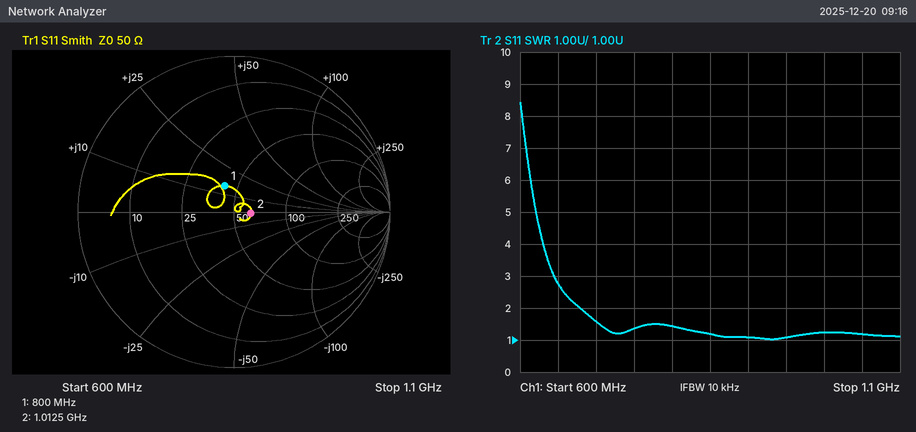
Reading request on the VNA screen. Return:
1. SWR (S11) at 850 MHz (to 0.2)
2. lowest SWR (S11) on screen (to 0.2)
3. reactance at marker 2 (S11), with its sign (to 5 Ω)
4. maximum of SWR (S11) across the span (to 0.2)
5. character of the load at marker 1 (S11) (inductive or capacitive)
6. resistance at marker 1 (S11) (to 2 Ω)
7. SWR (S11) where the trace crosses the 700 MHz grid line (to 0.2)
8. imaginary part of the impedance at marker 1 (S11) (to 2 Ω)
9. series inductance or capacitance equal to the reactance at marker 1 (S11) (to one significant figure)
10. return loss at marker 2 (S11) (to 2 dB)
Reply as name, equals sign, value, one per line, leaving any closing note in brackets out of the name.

SWR (S11) at 850 MHz = 1.2
lowest SWR (S11) on screen = 1.0
reactance at marker 2 (S11), with its sign = 0 Ω
maximum of SWR (S11) across the span = 8.4
character of the load at marker 1 (S11) = inductive
resistance at marker 1 (S11) = 42 Ω
SWR (S11) where the trace crosses the 700 MHz grid line = 1.6
imaginary part of the impedance at marker 1 (S11) = +14 Ω
series inductance or capacitance equal to the reactance at marker 1 (S11) = 3 nH
return loss at marker 2 (S11) = 20 dB
